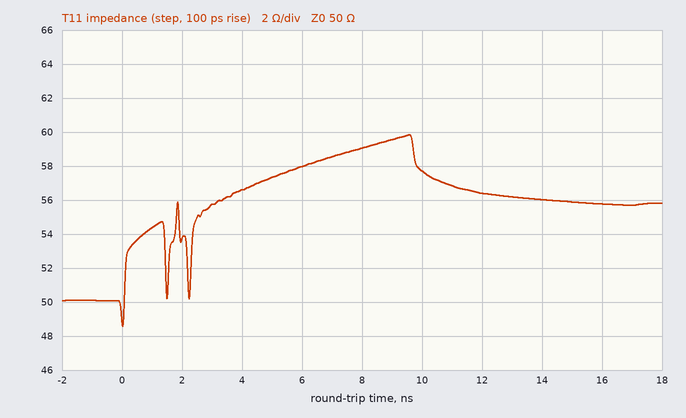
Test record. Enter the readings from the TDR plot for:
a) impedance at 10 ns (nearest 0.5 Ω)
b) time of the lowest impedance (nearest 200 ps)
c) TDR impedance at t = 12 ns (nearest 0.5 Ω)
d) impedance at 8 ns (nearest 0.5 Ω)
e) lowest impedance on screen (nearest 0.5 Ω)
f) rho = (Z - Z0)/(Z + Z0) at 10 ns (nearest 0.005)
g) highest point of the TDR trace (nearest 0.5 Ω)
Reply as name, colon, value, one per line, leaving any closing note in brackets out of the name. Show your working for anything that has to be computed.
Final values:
impedance at 10 ns: 57.5 Ω
time of the lowest impedance: 0.0 ns
TDR impedance at t = 12 ns: 56.5 Ω
impedance at 8 ns: 59.0 Ω
lowest impedance on screen: 48.5 Ω
rho = (Z - Z0)/(Z + Z0) at 10 ns: (57.5 − 50)/(57.5 + 50) ≈ +0.070
highest point of the TDR trace: 60.0 Ω
